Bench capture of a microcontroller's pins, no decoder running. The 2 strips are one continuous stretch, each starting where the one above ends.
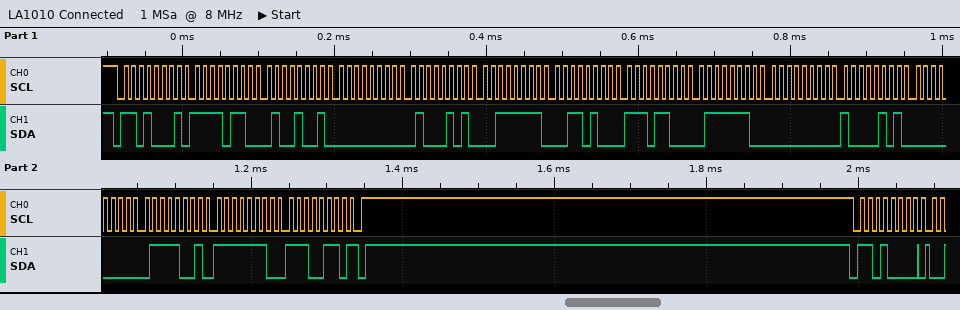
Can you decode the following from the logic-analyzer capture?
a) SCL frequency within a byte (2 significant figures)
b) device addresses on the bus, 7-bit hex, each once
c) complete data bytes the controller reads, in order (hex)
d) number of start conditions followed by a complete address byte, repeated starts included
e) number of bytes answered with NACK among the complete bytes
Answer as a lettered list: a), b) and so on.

a) 100 kHz
b) 0x68
c) F6 49 00 45 3F 34 EC 7E 00 85 00 79 FE E6
d) 2
e) 1
